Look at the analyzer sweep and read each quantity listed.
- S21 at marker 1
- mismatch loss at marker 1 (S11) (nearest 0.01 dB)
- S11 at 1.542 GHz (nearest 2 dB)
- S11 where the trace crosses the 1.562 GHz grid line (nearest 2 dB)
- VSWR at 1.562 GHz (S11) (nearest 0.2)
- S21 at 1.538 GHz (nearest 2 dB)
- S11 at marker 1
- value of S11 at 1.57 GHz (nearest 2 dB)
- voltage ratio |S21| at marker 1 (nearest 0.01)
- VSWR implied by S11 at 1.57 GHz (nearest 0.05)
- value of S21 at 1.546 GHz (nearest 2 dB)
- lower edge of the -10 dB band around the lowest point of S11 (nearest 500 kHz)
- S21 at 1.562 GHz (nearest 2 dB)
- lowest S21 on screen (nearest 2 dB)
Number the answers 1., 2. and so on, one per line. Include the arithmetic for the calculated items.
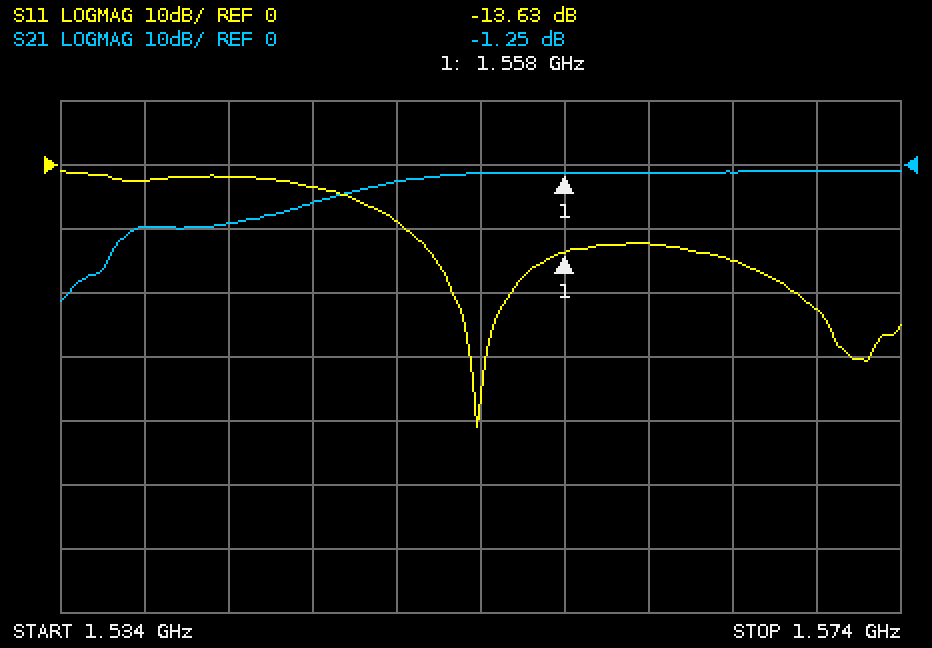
1. -1.25 dB
2. −10 log10(1 − 10^(-13.63/10)) ≈ 0.19 dB
3. -2 dB
4. -12 dB
5. |Γ| = 10^(-12/20) = 0.2512; VSWR = (1 + 0.2512)/(1 − 0.2512) ≈ 1.67, so 1.6 to the nearest 0.2
6. -10 dB
7. -13.63 dB
8. -22 dB
9. 10^(-1.25/20) ≈ 0.87
10. |Γ| = 10^(-22/20) = 0.0794; VSWR = (1 + 0.0794)/(1 − 0.0794) ≈ 1.17, so 1.15 to the nearest 0.05
11. -6 dB
12. 1.5505 GHz
13. -2 dB
14. -22 dB
